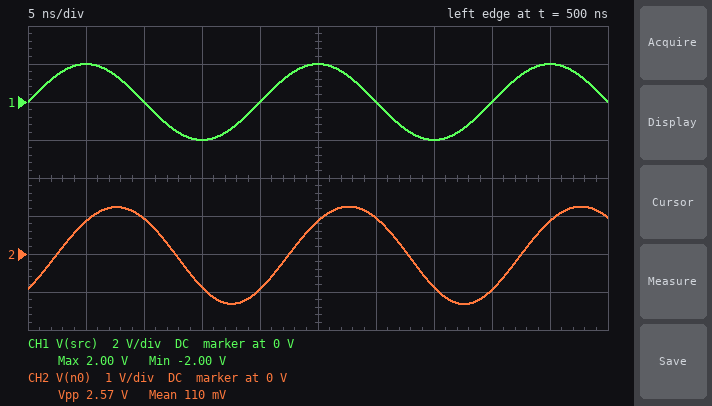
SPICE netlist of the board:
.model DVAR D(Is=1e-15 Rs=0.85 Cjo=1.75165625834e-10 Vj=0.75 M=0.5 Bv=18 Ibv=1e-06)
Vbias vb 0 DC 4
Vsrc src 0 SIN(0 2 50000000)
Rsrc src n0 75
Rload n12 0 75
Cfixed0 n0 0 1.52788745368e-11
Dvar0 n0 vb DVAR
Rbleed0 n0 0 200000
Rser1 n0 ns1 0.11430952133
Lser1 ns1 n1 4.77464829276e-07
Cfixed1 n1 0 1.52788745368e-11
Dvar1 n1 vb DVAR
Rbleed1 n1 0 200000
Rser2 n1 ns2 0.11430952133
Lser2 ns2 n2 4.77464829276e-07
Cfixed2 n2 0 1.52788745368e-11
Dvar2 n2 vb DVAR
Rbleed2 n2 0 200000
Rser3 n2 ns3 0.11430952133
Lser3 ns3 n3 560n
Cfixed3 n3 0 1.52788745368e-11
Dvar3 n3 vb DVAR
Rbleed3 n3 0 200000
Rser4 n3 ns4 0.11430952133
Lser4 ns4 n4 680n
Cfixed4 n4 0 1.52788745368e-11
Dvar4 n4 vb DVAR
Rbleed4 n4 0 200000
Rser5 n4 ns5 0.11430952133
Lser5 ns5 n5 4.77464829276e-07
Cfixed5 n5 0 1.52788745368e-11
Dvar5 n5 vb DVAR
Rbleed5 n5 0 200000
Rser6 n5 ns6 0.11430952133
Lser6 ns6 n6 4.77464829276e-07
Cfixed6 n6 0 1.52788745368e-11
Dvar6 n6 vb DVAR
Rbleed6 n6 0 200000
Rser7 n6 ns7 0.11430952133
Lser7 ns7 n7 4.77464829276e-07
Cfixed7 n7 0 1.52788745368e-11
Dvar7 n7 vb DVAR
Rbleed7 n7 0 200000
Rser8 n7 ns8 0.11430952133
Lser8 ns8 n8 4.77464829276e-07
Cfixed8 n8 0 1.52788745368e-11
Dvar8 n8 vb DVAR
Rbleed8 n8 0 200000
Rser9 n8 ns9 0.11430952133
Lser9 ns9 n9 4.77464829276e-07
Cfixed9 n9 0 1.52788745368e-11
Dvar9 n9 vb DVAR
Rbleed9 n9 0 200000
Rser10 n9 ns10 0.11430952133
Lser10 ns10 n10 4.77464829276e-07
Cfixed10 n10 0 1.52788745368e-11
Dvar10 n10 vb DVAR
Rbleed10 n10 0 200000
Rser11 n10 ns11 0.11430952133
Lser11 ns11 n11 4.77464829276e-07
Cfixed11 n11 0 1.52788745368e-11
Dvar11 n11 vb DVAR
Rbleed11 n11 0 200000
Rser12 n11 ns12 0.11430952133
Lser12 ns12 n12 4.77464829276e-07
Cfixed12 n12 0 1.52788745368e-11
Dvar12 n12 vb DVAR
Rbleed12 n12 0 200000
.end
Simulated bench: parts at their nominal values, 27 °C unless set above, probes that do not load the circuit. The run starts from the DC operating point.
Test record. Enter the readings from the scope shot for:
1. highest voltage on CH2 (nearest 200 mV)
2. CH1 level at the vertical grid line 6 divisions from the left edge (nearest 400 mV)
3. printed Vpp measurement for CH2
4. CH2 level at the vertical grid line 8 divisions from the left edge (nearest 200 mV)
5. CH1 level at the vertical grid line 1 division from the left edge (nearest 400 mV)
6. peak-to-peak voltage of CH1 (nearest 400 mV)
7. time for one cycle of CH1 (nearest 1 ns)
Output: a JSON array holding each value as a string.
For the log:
["1.2 V", "0 V", "2.57 V", "-1.0 V", "2.0 V", "4.0 V", "20 ns"]
